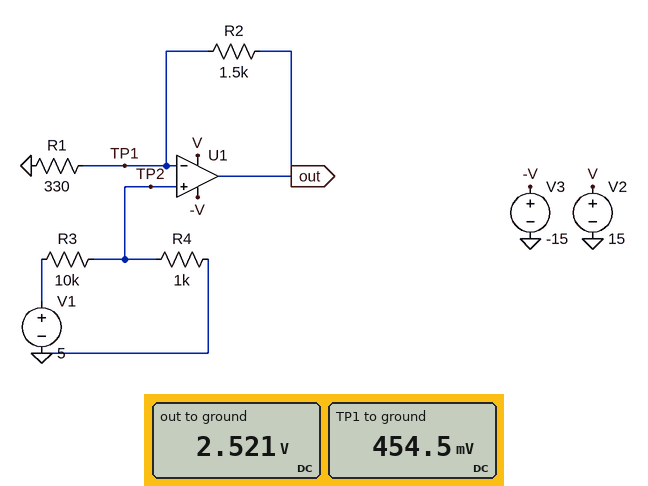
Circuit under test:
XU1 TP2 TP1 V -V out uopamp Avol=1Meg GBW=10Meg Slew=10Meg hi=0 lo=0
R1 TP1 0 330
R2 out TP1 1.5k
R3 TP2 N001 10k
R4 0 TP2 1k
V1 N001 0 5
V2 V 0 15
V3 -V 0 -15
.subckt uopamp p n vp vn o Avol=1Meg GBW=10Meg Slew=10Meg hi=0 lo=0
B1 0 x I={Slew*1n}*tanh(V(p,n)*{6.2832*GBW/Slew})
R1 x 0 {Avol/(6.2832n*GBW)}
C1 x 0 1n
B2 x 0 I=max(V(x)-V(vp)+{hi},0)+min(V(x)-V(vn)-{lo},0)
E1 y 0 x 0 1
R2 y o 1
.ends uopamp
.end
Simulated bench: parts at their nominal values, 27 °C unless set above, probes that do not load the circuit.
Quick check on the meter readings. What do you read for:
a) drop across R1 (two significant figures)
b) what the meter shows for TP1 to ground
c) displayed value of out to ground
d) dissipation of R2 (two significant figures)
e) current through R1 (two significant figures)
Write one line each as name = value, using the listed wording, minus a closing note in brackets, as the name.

drop across R1 = 450 mV
what the meter shows for TP1 to ground = 454.5 mV
displayed value of out to ground = 2.521 V
dissipation of R2 = 2.8 mW
current through R1 = 1.4 mA
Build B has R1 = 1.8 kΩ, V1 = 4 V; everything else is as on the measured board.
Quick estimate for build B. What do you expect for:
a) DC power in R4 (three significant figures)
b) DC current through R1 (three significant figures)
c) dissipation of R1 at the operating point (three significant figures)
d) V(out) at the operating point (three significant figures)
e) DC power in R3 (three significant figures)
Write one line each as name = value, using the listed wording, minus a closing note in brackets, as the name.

DC power in R4 = 132 µW
DC current through R1 = 202 µA
dissipation of R1 at the operating point = 73.5 µW
V(out) at the operating point = 667 mV
DC power in R3 = 1.32 mW
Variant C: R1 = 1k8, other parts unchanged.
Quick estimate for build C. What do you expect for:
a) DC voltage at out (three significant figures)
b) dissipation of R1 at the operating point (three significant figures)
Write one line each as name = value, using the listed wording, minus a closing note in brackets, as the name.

DC voltage at out = 833 mV
dissipation of R1 at the operating point = 115 µW
